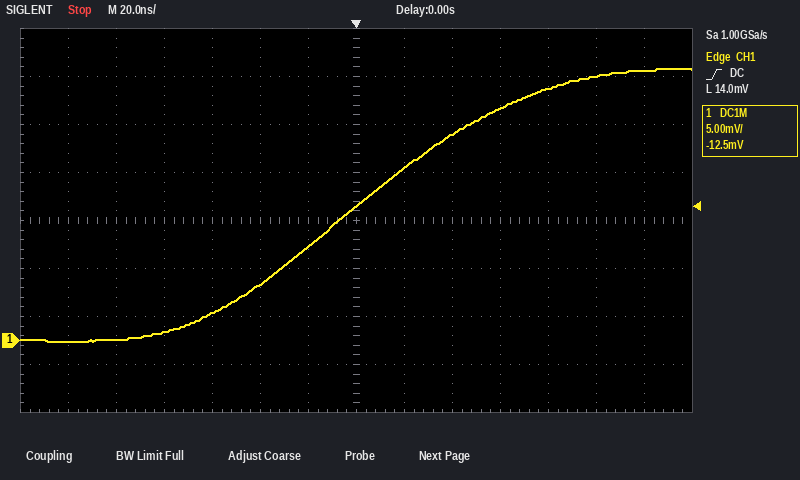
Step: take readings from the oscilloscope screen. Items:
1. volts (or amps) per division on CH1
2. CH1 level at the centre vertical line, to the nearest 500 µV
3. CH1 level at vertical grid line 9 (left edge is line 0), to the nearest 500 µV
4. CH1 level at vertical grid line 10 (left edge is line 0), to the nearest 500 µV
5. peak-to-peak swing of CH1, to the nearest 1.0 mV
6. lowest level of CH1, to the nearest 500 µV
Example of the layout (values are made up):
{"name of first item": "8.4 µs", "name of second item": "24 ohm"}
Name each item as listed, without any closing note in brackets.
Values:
{"volts (or amps) per division on CH1": "5 mV", "CH1 level at the centre vertical line, to the nearest 500 µV": "14.0 mV", "CH1 level at vertical grid line 9 (left edge is line 0), to the nearest 500 µV": "21.5 mV", "CH1 level at vertical grid line 10 (left edge is line 0), to the nearest 500 µV": "24.0 mV", "peak-to-peak swing of CH1, to the nearest 1.0 mV": "28.0 mV", "lowest level of CH1, to the nearest 500 µV": "0.0 mV"}
